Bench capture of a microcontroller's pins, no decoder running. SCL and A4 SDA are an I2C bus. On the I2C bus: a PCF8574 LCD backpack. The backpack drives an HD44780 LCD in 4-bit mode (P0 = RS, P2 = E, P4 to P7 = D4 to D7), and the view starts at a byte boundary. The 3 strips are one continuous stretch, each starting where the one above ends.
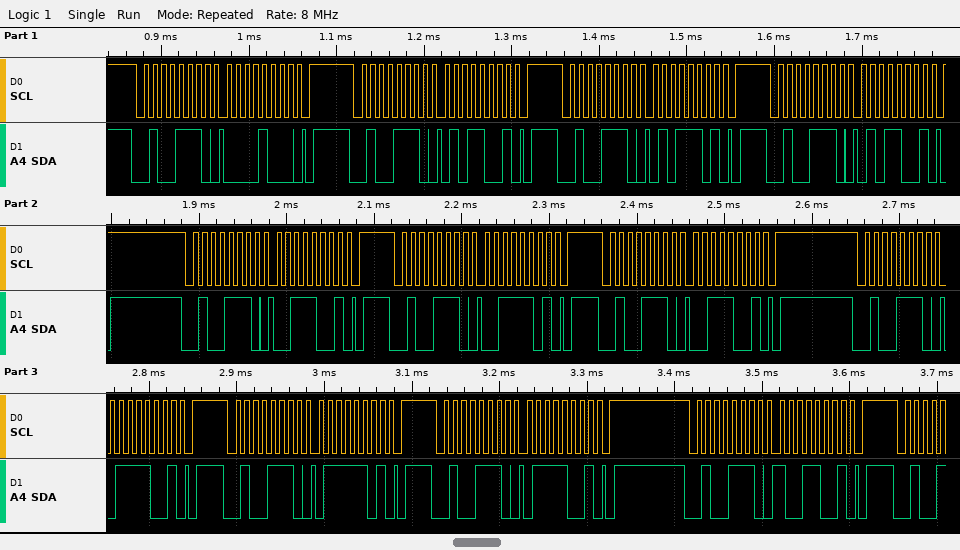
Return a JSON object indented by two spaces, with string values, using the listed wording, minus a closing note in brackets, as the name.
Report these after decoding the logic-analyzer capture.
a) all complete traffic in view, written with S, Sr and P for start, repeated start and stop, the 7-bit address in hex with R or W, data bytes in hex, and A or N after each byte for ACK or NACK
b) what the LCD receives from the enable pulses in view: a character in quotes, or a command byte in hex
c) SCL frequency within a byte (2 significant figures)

{
  "all complete traffic in view, written with S, Sr and P for start, repeated start and stop, the 7-bit address in hex with R or W, data bytes in hex, and A or N after each byte for ACK or NACK": "S 27W A 08 A P S 27W A 59 A P S 27W A 5D A P S 27W A 59 A P S 27W A 39 A P S 27W A 3D A P S 27W A 39 A P S 27W A 79 A P S 27W A 7D A P S 27W A 79 A P S 27W A 99 A P",
  "what the LCD receives from the enable pulses in view: a character in quotes, or a command byte in hex": "'S'",
  "SCL frequency within a byte": "100 kHz"
}
